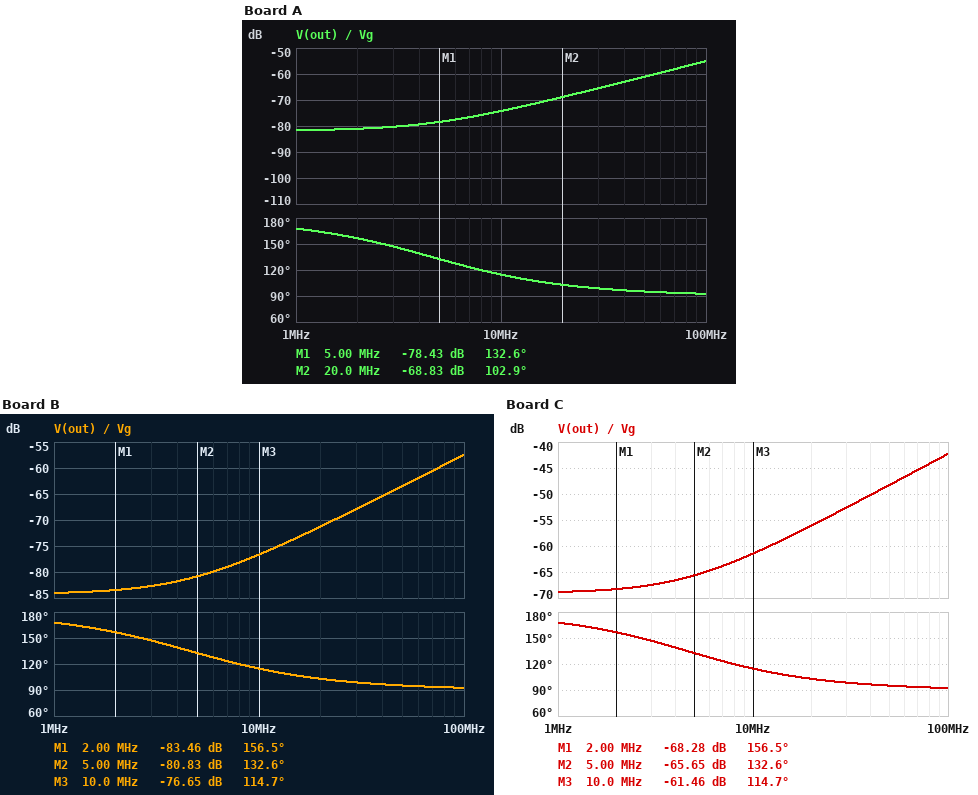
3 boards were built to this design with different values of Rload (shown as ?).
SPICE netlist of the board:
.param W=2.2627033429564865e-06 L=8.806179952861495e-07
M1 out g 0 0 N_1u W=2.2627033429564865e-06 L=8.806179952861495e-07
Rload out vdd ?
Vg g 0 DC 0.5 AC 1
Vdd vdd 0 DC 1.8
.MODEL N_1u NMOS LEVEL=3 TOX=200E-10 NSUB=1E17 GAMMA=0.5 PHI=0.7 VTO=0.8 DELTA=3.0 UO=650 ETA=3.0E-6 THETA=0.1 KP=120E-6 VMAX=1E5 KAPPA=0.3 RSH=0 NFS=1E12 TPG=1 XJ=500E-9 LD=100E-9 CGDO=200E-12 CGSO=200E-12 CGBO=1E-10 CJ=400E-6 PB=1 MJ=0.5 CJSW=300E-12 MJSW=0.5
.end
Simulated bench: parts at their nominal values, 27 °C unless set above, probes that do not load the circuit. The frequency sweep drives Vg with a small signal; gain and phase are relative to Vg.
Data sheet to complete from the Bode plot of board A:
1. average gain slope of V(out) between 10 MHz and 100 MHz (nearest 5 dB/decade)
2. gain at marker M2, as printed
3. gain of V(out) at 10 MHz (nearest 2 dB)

20 dB/decade
-68.83 dB
-74 dB
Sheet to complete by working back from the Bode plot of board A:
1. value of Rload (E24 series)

6.2 kΩ
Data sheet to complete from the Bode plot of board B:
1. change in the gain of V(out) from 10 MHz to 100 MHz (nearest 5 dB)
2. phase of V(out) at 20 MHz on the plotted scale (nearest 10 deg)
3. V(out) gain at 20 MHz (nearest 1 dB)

20 dB
100 deg
-71 dB
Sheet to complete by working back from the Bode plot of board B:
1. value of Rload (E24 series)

4.7 kΩ
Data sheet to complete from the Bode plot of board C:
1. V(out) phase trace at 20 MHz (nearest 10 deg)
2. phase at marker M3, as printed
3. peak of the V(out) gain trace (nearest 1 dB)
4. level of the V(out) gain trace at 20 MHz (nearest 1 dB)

100 deg
114.7 deg
-42 dB
-56 dB
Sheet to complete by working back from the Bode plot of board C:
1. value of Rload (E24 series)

27 kΩ
